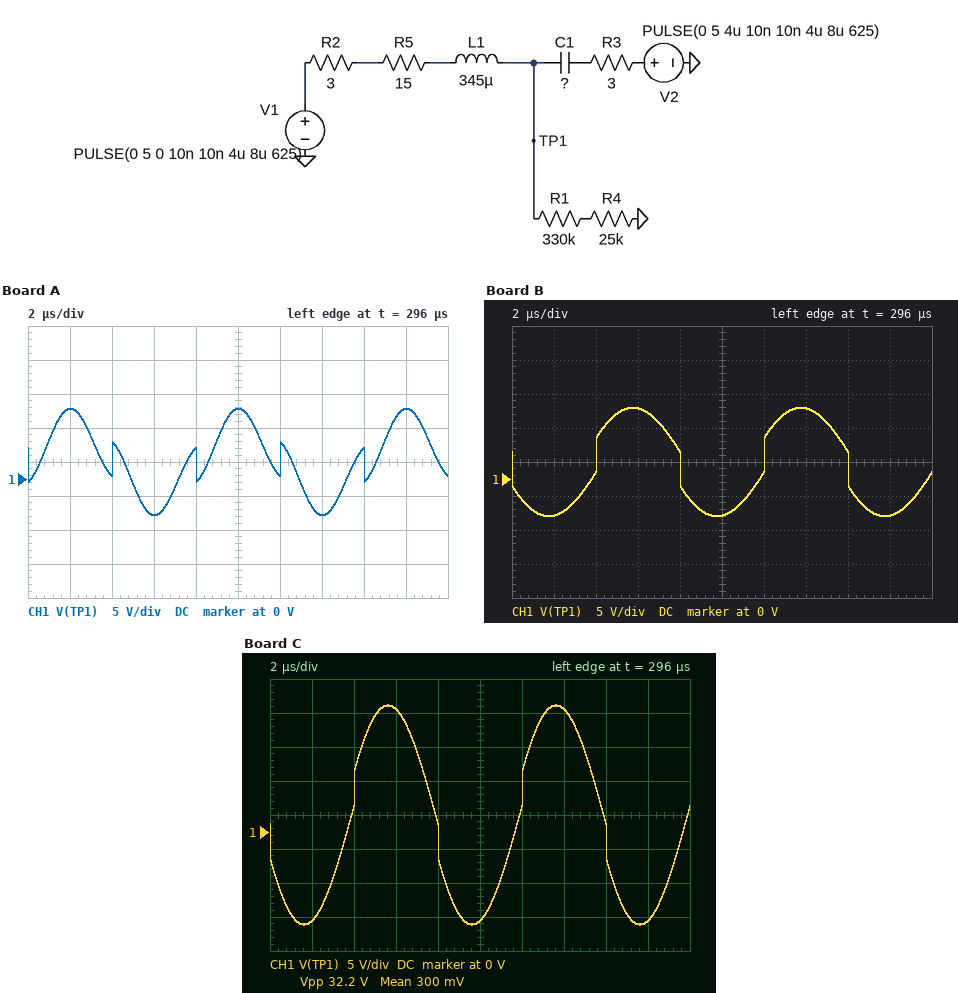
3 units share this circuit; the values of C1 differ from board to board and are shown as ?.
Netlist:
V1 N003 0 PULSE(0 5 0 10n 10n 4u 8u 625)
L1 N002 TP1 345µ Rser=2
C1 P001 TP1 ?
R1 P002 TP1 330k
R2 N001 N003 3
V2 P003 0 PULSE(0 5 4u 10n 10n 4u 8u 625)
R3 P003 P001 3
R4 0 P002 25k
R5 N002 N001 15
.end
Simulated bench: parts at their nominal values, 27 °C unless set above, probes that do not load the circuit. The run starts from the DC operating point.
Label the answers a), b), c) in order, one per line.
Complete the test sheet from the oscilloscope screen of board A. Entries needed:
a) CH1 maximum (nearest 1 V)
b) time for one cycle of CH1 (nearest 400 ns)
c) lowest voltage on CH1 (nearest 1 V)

a) 10 V
b) 8.0 µs
c) -5 V
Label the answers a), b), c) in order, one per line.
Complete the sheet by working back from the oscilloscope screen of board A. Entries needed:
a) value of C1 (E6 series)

a) 1.5 nF
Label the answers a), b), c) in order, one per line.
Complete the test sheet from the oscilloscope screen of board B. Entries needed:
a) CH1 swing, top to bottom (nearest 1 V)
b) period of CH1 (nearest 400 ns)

a) 16 V
b) 8.0 µs
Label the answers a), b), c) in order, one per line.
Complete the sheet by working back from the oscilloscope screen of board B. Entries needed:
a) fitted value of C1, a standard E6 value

a) 10 nF
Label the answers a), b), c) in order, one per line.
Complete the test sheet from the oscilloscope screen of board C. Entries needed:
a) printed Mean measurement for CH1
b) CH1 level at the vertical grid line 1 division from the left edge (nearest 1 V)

a) 300 mV
b) -13 V
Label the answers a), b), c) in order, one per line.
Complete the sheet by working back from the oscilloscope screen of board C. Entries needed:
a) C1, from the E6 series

a) 6.8 nF
